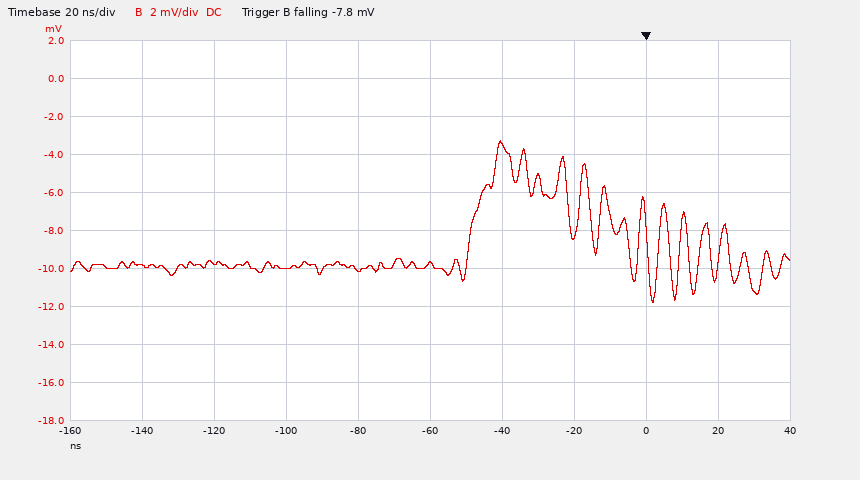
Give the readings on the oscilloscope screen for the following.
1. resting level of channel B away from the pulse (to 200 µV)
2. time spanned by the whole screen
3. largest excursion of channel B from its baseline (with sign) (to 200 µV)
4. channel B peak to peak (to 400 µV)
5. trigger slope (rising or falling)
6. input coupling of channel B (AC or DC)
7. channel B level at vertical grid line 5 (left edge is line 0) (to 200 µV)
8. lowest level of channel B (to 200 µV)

-9.8 mV
200 ns
+6.6 mV
8.4 mV
falling
DC
-9.8 mV
-11.8 mV
